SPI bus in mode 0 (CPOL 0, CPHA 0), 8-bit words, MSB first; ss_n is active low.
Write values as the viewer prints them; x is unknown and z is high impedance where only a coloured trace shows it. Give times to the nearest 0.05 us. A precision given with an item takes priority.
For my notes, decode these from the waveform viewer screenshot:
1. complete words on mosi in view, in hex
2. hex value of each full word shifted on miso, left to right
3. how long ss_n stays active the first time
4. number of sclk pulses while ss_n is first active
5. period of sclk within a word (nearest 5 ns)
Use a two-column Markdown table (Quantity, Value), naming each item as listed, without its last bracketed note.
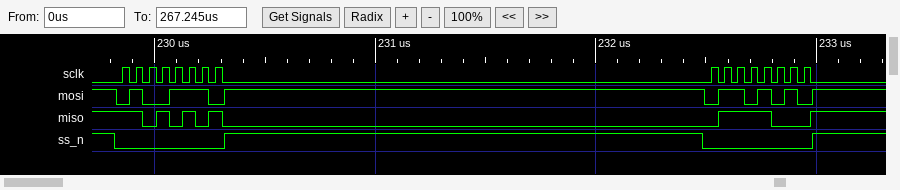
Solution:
| Quantity | Value |
|---|---|
| complete words on mosi in view, in hex | 4E, 6A |
| hex value of each full word shifted on miso, left to right | D5, 78 |
| how long ss_n stays active the first time | 0.5 us |
| number of sclk pulses while ss_n is first active | 8 |
| period of sclk within a word | 60 ns |
